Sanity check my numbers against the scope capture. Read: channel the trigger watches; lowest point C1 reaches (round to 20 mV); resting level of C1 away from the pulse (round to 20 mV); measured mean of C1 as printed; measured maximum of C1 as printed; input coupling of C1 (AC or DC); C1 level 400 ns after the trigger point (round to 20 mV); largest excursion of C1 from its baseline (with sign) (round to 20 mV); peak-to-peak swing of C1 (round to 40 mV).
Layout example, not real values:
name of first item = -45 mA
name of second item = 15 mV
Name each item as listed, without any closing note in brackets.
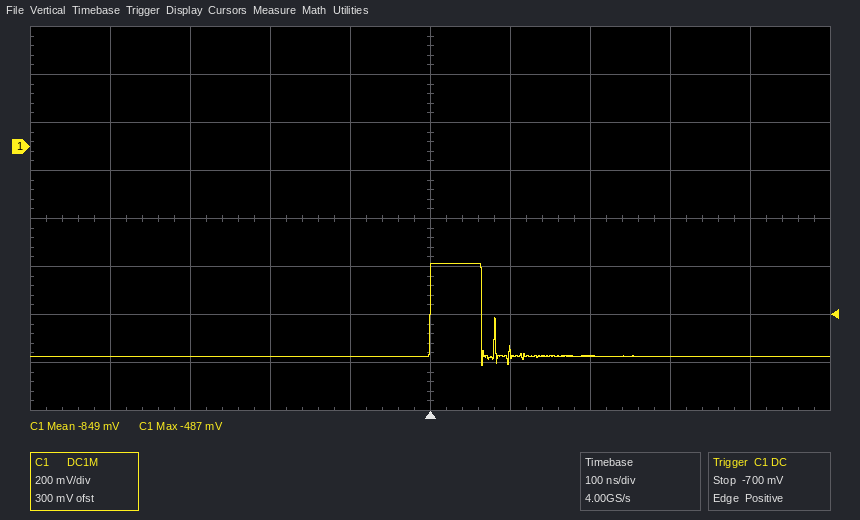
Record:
channel the trigger watches = C1
lowest point C1 reaches = -920 mV
resting level of C1 away from the pulse = -880 mV
measured mean of C1 as printed = -849 mV
measured maximum of C1 as printed = -487 mV
input coupling of C1 = DC
C1 level 400 ns after the trigger point = -880 mV
largest excursion of C1 from its baseline (with sign) = +380 mV
peak-to-peak swing of C1 = 440 mV
